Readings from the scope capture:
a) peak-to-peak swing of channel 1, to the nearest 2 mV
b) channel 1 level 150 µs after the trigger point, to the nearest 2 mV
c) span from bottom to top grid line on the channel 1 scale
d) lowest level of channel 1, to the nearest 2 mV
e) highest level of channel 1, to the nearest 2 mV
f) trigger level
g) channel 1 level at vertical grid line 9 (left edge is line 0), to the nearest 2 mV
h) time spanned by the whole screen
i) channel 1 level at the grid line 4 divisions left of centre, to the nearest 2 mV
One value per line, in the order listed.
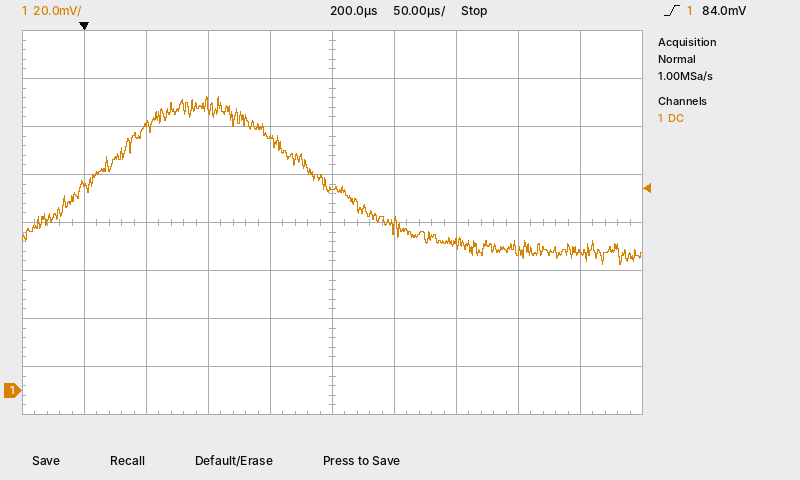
70 mV
106 mV
160 mV
52 mV
122 mV
84.0 mV
58 mV
500 µs
86 mV
